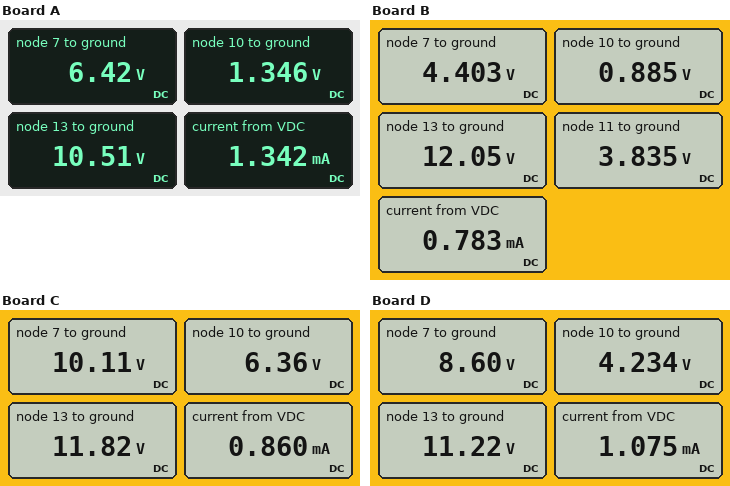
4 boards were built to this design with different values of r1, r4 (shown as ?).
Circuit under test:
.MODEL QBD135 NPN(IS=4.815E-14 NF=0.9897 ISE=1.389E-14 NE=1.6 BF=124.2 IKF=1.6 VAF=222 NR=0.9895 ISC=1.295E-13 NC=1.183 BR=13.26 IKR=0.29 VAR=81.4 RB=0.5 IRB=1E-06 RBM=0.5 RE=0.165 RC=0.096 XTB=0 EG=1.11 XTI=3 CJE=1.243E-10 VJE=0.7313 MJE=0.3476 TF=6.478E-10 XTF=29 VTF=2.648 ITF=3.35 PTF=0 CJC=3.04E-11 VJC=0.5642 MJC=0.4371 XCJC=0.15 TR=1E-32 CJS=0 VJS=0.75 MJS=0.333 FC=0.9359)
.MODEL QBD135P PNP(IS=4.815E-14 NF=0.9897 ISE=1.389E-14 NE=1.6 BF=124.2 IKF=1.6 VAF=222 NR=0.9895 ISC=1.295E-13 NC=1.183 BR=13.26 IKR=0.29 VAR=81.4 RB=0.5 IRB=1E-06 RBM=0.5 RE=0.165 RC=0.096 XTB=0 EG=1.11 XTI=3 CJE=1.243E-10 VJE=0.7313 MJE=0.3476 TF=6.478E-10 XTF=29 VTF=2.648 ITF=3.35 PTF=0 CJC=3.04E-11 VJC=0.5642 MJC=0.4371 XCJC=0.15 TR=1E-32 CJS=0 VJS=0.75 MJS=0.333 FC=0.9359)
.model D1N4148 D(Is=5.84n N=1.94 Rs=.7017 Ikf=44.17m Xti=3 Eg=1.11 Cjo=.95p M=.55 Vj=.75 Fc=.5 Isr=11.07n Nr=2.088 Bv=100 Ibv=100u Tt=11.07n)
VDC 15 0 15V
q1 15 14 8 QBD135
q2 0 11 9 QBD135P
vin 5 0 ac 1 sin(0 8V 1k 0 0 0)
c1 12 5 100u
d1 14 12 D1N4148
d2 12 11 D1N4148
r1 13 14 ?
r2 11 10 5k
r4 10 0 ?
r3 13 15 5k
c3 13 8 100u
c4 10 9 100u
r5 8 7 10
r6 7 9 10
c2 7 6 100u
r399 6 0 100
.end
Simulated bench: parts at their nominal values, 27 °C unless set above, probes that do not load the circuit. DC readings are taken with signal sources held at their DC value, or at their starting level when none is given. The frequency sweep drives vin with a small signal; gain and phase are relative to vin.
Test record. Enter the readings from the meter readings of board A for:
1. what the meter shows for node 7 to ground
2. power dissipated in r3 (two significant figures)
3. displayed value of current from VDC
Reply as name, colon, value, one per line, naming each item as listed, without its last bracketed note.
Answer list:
what the meter shows for node 7 to ground: 6.42 V
power dissipated in r3: 4.0 mW
displayed value of current from VDC: 1.342 mA
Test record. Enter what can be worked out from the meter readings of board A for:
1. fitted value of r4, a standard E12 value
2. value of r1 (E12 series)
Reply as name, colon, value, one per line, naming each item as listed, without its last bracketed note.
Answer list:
fitted value of r4, a standard E12 value: 1.5 kΩ
value of r1: 3.9 kΩ
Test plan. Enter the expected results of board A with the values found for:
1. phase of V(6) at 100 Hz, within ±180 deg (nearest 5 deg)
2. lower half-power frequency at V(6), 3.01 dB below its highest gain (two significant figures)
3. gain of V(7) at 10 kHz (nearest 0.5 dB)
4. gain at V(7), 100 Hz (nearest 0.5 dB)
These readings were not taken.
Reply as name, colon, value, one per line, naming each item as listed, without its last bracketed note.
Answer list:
phase of V(6) at 100 Hz, within ±180 deg: 5 deg
lower half-power frequency at V(6), 3.01 dB below its highest gain: 21 Hz
gain of V(7) at 10 kHz: -2.5 dB
gain at V(7), 100 Hz: -2.5 dB
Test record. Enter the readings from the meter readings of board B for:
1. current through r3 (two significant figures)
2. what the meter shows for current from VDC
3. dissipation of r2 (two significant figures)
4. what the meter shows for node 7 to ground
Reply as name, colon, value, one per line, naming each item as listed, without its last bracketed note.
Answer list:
current through r3: 590 µA
what the meter shows for current from VDC: 0.783 mA
dissipation of r2: 1.7 mW
what the meter shows for node 7 to ground: 4.403 V
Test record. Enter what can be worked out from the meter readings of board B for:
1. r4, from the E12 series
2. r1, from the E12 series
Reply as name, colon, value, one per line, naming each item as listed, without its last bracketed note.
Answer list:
r4, from the E12 series: 1.5 kΩ
r1, from the E12 series: 12 kΩ
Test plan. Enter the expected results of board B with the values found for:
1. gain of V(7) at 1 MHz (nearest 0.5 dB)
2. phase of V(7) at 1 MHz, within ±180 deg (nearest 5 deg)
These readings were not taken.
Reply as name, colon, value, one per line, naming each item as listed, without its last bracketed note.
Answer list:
gain of V(7) at 1 MHz: -5.0 dB
phase of V(7) at 1 MHz, within ±180 deg: 0 deg
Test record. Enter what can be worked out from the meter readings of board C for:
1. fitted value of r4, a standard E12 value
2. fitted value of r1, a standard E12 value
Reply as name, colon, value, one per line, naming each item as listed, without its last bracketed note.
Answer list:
fitted value of r4, a standard E12 value: 10 kΩ
fitted value of r1, a standard E12 value: 1.8 kΩ
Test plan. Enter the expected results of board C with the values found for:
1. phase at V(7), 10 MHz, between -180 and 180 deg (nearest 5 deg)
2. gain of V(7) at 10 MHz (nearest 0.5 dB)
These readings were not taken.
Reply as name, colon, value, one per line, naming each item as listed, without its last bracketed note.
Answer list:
phase at V(7), 10 MHz, between -180 and 180 deg: 10 deg
gain of V(7) at 10 MHz: -4.0 dB
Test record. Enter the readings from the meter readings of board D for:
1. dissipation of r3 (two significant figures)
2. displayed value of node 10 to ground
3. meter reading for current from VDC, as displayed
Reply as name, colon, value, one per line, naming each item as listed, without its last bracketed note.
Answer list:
dissipation of r3: 2.9 mW
displayed value of node 10 to ground: 4.234 V
meter reading for current from VDC, as displayed: 1.075 mA
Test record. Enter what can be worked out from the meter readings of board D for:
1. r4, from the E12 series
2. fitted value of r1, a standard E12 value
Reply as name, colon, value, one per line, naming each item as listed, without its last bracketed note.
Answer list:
r4, from the E12 series: 5.6 kΩ
fitted value of r1, a standard E12 value: 2.7 kΩ
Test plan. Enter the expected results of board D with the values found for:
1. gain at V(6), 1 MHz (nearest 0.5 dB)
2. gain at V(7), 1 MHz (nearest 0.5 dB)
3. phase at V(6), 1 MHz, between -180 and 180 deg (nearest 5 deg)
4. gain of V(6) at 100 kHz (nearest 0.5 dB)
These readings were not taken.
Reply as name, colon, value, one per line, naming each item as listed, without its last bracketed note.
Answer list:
gain at V(6), 1 MHz: -3.5 dB
gain at V(7), 1 MHz: -3.5 dB
phase at V(6), 1 MHz, between -180 and 180 deg: 0 deg
gain of V(6) at 100 kHz: -3.5 dB
